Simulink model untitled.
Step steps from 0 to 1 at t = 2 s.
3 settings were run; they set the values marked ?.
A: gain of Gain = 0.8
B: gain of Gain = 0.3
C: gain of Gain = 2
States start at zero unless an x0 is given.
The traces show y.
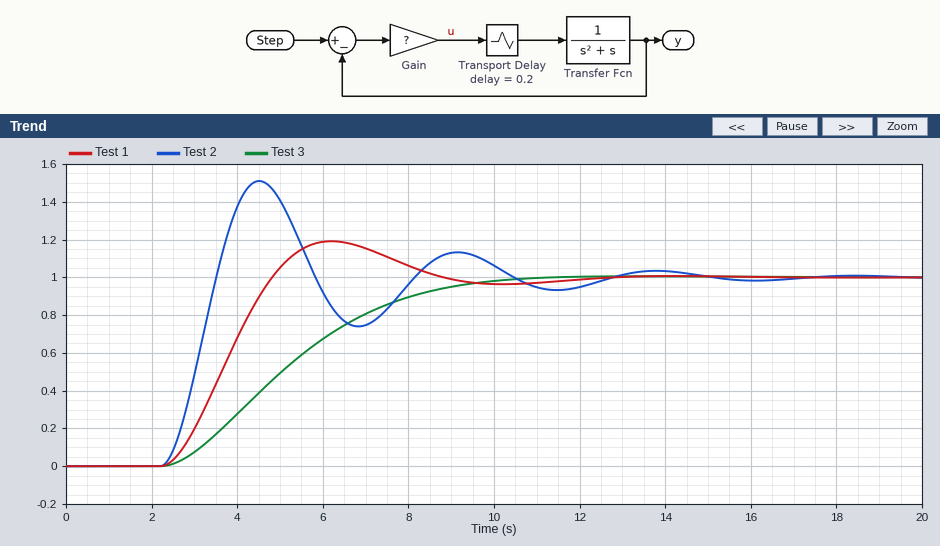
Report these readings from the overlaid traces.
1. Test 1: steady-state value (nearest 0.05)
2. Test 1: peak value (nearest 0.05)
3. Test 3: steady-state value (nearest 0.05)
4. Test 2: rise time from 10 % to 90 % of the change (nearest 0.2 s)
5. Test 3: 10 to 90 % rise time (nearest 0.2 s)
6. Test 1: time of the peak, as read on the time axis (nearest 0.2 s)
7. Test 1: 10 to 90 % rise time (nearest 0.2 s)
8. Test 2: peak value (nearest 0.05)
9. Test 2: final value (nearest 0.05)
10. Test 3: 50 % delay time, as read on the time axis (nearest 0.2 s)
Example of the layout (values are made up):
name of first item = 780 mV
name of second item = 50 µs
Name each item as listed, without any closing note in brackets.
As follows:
Test 1: steady-state value = 1.00
Test 1: peak value = 1.20
Test 3: steady-state value = 1.00
Test 2: rise time from 10 % to 90 % of the change = 0.8 s
Test 3: 10 to 90 % rise time = 5.0 s
Test 1: time of the peak, as read on the time axis = 6.2 s
Test 1: 10 to 90 % rise time = 1.8 s
Test 2: peak value = 1.50
Test 2: final value = 1.00
Test 3: 50 % delay time, as read on the time axis = 5.0 s
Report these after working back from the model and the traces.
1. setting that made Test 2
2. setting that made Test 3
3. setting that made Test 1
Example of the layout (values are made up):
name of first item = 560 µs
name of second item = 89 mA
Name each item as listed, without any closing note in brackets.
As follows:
setting that made Test 2 = C
setting that made Test 3 = B
setting that made Test 1 = A
